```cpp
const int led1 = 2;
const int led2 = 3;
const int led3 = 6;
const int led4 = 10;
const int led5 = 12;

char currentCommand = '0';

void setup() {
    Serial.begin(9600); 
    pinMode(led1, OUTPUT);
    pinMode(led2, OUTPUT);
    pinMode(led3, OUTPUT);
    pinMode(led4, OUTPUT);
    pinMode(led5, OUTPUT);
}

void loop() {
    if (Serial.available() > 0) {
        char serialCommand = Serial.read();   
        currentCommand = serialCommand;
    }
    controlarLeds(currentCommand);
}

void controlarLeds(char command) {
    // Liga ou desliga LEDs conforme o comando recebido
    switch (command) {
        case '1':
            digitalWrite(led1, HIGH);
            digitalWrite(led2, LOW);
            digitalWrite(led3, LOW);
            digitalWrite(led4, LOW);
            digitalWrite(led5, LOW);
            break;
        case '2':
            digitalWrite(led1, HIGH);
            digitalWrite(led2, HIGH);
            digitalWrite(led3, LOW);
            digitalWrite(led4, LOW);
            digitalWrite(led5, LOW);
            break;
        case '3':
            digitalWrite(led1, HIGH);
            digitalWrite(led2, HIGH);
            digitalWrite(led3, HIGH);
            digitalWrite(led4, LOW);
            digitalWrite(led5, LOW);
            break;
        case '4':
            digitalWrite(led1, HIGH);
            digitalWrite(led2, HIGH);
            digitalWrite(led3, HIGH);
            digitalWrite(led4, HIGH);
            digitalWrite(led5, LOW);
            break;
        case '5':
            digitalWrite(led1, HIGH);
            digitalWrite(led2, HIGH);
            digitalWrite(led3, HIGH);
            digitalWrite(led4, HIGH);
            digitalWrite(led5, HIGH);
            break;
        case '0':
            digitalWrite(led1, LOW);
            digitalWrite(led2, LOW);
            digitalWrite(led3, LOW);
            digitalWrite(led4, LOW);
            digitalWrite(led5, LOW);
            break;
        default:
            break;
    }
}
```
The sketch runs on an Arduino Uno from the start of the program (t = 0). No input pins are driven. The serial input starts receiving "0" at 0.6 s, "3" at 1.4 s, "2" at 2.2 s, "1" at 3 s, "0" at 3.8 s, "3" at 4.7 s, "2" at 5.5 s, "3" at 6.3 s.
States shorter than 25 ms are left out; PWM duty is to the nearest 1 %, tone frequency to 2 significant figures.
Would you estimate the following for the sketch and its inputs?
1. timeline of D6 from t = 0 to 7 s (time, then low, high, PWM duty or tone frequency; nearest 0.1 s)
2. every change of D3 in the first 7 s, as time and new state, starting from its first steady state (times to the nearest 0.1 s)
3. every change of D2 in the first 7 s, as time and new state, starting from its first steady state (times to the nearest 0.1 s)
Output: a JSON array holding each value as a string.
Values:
["0 s low; 1.4 s high; 2.2 s low; 4.7 s high; 5.5 s low; 6.3 s high", "0 s low; 1.4 s high; 3 s low; 4.7 s high", "0 s low; 1.4 s high; 3.8 s low; 4.7 s high"]
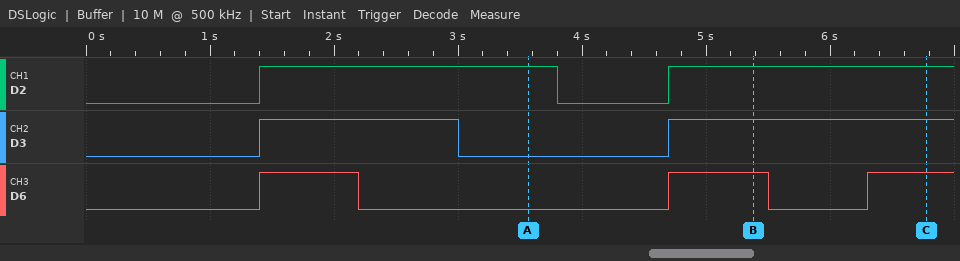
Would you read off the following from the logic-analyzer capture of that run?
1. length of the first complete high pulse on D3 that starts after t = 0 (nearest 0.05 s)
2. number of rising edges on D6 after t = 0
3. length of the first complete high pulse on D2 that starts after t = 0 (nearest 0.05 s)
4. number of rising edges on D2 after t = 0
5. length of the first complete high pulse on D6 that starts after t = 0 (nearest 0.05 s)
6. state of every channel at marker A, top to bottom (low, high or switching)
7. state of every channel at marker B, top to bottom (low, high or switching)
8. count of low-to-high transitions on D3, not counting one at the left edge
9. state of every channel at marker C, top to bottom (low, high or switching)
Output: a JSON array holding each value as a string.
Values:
["1.60 s", "3", "2.40 s", "2", "0.80 s", "D2 high, D3 low, D6 low", "D2 high, D3 high, D6 high", "2", "D2 high, D3 high, D6 high"]
